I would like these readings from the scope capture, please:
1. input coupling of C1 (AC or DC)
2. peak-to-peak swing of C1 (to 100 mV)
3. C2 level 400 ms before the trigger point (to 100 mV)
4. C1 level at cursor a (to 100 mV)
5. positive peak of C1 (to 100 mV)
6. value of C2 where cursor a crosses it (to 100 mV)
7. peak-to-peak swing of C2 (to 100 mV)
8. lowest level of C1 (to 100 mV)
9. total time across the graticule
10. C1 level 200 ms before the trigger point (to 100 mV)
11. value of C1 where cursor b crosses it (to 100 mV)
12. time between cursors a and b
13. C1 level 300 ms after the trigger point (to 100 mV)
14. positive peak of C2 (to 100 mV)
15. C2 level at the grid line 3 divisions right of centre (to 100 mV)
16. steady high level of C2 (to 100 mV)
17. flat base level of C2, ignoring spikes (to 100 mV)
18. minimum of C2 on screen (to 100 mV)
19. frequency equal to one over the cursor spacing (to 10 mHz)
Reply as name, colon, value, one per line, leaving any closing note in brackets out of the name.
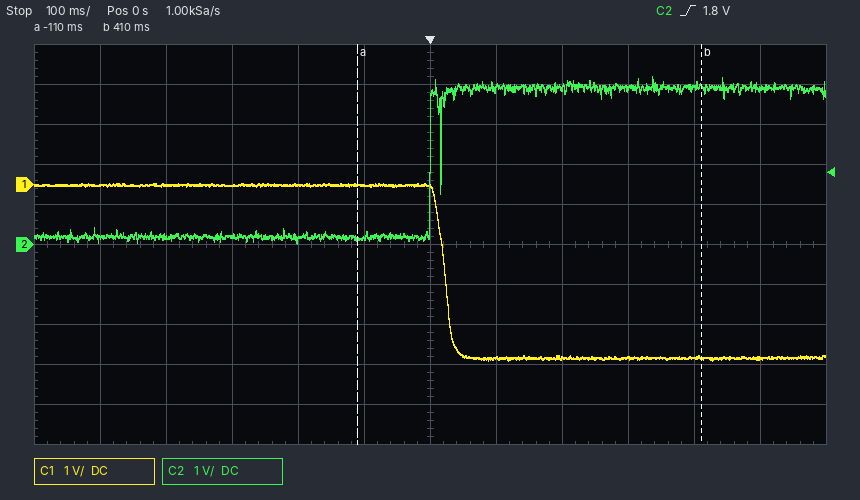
input coupling of C1: DC
peak-to-peak swing of C1: 4.4 V
C2 level 400 ms before the trigger point: 200 mV
C1 level at cursor a: 0.0 V
positive peak of C1: 0.0 V
value of C2 where cursor a crosses it: 200 mV
peak-to-peak swing of C2: 4.2 V
lowest level of C1: -4.4 V
total time across the graticule: 1.2 s
C1 level 200 ms before the trigger point: 0.0 V
value of C1 where cursor b crosses it: -4.3 V
time between cursors a and b: 520 ms
C1 level 300 ms after the trigger point: -4.3 V
positive peak of C2: 4.2 V
C2 level at the grid line 3 divisions right of centre: 3.9 V
steady high level of C2: 3.9 V
flat base level of C2, ignoring spikes: 200 mV
minimum of C2 on screen: 0.0 V
frequency equal to one over the cursor spacing: 1.92 Hz
